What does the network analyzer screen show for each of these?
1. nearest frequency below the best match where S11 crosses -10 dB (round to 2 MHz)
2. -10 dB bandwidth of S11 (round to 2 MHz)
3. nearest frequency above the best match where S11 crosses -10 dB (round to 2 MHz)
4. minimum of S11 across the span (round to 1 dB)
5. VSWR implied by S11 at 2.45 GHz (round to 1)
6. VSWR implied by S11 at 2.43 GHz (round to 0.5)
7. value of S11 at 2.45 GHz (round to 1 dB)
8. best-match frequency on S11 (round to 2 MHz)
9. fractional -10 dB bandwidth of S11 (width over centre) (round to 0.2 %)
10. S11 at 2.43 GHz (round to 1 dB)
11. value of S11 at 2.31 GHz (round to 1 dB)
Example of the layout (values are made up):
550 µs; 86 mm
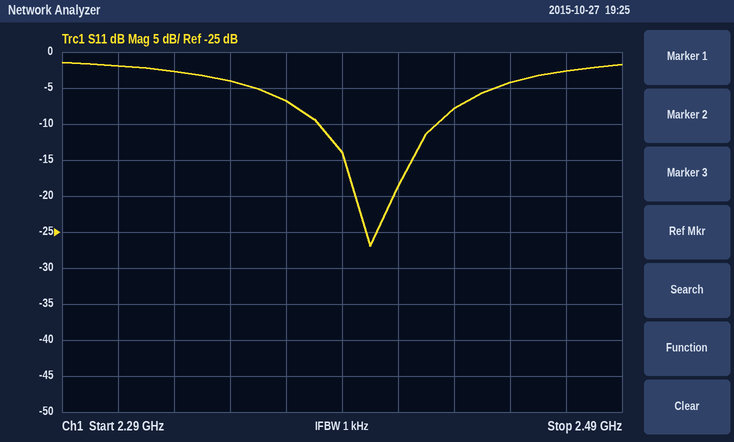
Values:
2.382 GHz; 42 MHz; 2.424 GHz; -27 dB; 4; 2.5; -4 dB; 2.400 GHz; 1.8 %; -8 dB; -2 dB
